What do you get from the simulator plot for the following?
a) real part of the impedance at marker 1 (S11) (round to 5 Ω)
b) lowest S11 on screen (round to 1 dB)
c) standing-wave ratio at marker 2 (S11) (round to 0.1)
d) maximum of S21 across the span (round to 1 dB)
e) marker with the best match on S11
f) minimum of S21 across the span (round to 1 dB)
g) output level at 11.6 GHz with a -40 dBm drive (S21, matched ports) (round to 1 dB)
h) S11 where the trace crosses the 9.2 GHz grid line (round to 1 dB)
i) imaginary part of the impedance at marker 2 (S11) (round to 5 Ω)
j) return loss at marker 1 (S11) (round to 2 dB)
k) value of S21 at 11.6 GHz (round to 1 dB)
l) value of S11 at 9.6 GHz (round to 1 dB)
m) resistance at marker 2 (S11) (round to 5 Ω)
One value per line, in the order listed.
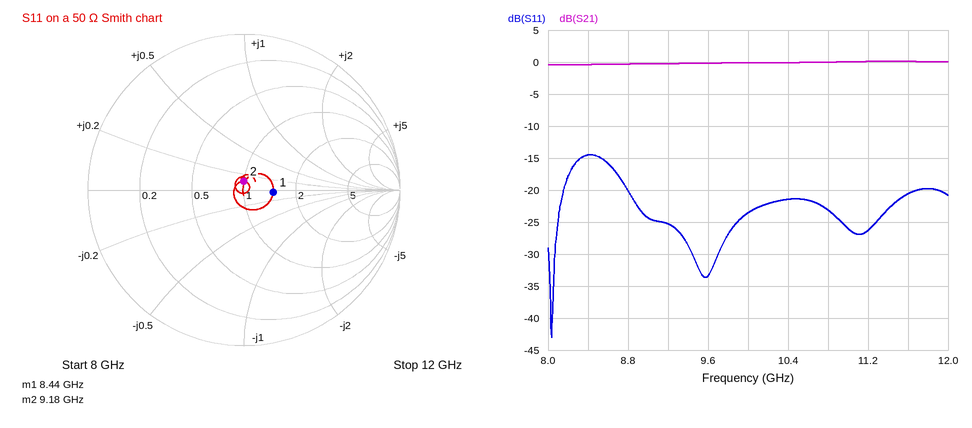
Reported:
75 Ω
-43 dB
1.1
0 dB
marker 2
0 dB
-40 dBm
-25 dB
+5 Ω
14 dB
0 dB
-33 dB
50 Ω
